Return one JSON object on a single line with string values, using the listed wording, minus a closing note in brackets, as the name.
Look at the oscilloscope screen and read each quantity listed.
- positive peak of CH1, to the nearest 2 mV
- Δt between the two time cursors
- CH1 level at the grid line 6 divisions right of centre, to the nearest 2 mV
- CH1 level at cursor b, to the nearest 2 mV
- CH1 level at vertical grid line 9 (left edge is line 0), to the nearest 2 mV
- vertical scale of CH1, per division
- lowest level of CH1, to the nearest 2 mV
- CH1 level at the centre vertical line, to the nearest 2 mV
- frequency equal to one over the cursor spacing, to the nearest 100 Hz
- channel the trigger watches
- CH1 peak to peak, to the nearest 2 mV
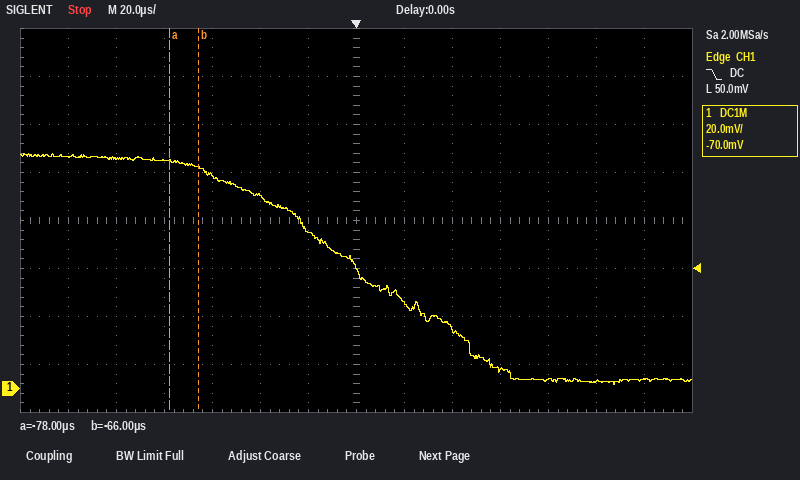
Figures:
{"positive peak of CH1, to the nearest 2 mV": "98 mV", "Δt between the two time cursors": "12 µs", "CH1 level at the grid line 6 divisions right of centre, to the nearest 2 mV": "4 mV", "CH1 level at cursor b, to the nearest 2 mV": "92 mV", "CH1 level at vertical grid line 9 (left edge is line 0), to the nearest 2 mV": "24 mV", "vertical scale of CH1, per division": "20 mV", "lowest level of CH1, to the nearest 2 mV": "2 mV", "CH1 level at the centre vertical line, to the nearest 2 mV": "50 mV", "frequency equal to one over the cursor spacing, to the nearest 100 Hz": "83.3 kHz", "channel the trigger watches": "CH1", "CH1 peak to peak, to the nearest 2 mV": "96 mV"}
